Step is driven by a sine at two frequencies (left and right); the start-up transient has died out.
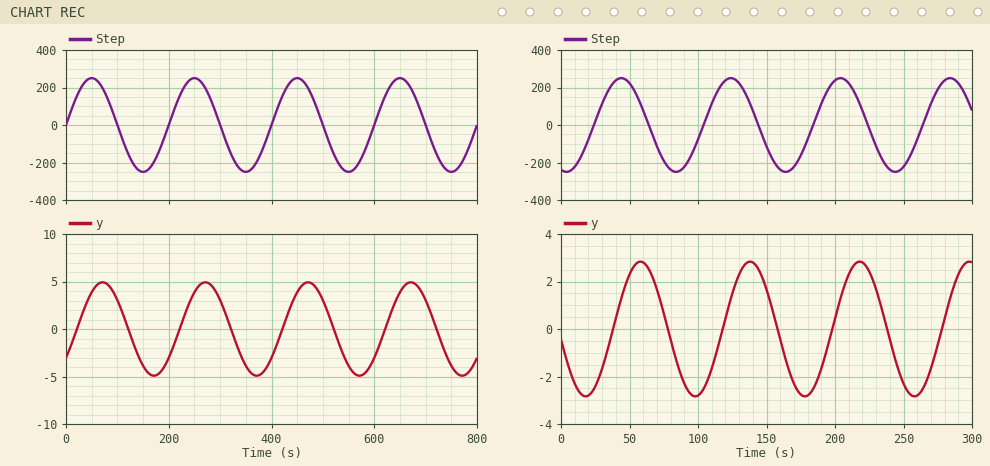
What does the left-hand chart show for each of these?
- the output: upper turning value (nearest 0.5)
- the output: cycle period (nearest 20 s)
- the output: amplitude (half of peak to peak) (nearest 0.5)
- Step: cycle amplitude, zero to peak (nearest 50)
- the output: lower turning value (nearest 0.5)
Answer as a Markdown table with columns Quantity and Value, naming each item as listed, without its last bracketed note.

| Quantity | Value |
|---|---|
| the output: upper turning value | 5.0 |
| the output: cycle period | 200 s |
| the output: amplitude (half of peak to peak) | 5.0 |
| Step: cycle amplitude, zero to peak | 250 |
| the output: lower turning value | -5.0 |
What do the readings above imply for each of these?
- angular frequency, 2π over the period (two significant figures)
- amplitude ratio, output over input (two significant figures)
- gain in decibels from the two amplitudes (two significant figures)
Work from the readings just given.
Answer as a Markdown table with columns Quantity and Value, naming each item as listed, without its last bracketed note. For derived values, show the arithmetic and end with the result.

| Quantity | Value |
|---|---|
| angular frequency, 2π over the period | 2π / 200 = 0.031 rad/s |
| amplitude ratio, output over input | 5 / 250 = 0.020 |
| gain in decibels from the two amplitudes | 20 log10(5 / 250) = -34 dB |
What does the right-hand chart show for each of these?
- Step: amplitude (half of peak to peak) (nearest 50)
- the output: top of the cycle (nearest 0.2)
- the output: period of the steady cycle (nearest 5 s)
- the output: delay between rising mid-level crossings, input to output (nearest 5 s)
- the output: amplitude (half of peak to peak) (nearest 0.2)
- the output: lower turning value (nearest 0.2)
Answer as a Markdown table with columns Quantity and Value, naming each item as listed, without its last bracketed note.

| Quantity | Value |
|---|---|
| Step: amplitude (half of peak to peak) | 250 |
| the output: top of the cycle | 2.8 |
| the output: period of the steady cycle | 80 s |
| the output: delay between rising mid-level crossings, input to output | 15 s |
| the output: amplitude (half of peak to peak) | 2.8 |
| the output: lower turning value | -2.8 |
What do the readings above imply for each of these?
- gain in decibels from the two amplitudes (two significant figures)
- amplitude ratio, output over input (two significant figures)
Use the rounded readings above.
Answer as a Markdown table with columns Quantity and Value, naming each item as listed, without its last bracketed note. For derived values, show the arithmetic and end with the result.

| Quantity | Value |
|---|---|
| gain in decibels from the two amplitudes | 20 log10(2.8 / 250) = -39 dB |
| amplitude ratio, output over input | 2.8 / 250 = 0.011 |
